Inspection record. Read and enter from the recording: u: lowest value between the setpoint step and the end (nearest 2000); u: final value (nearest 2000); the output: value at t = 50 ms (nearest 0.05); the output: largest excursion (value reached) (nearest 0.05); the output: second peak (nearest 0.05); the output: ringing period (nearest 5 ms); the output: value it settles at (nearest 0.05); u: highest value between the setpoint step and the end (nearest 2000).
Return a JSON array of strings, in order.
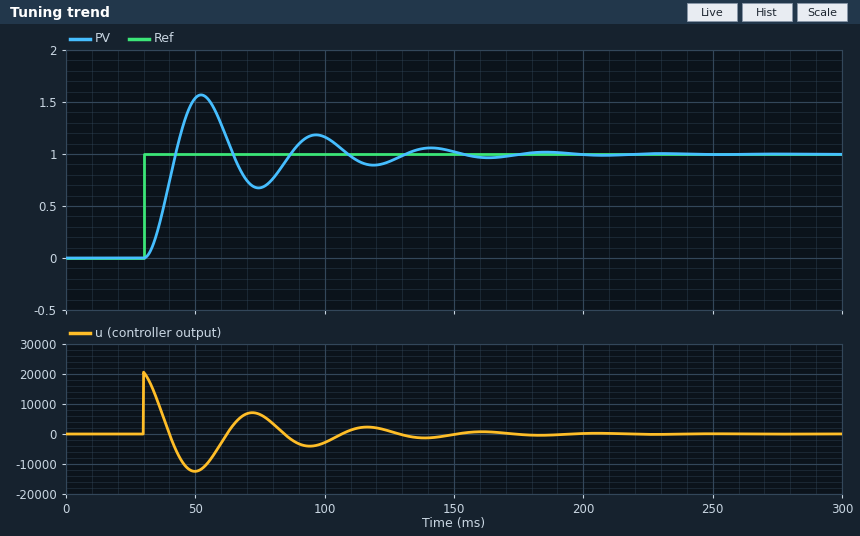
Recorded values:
["-12000", "0", "1.55", "1.55", "1.20", "45 ms", "1.00", "20000"]
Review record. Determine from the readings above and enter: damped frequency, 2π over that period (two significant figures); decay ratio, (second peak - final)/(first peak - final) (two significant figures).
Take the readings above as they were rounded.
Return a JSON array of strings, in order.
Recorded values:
["0.14 rad/ms", "0.36"]
